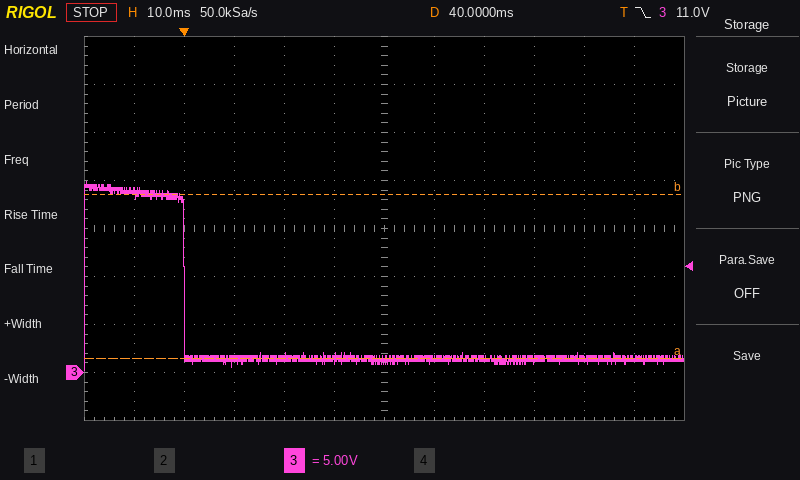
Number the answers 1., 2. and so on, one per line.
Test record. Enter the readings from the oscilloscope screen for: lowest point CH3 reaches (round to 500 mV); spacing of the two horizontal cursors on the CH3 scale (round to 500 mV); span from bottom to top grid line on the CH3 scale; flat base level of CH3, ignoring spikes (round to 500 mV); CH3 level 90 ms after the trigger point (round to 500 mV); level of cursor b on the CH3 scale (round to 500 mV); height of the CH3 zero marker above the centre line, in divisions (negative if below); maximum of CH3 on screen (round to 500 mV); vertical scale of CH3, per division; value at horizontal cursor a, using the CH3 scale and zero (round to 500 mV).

1. 0.0 V
2. 17.0 V
3. 40 V
4. 1.5 V
5. 1.5 V
6. 18.5 V
7. -3.0 div
8. 20.0 V
9. 5 V
10. 1.5 V
